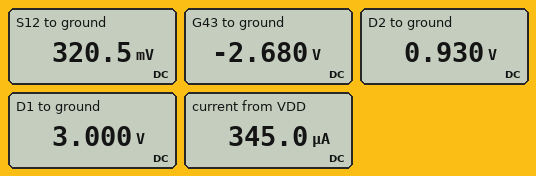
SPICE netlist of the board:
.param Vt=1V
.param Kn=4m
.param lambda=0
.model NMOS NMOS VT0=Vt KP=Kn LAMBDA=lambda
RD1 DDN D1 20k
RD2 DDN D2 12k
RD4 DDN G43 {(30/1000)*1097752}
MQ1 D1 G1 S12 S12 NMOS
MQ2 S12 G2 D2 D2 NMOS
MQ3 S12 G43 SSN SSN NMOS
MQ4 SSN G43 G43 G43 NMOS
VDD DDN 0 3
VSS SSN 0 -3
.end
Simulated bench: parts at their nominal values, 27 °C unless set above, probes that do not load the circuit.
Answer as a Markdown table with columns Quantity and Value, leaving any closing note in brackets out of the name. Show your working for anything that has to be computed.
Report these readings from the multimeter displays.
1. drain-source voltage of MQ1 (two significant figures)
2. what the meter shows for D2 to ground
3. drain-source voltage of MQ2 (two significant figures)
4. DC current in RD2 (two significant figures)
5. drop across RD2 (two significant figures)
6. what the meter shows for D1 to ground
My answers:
| Quantity | Value |
|---|---|
| drain-source voltage of MQ1 | 3 V - 320.5 mV = 2.7 V |
| what the meter shows for D2 to ground | 0.930 V |
| drain-source voltage of MQ2 | 320.5 mV - 930 mV = -610 mV |
| DC current in RD2 | (3 V - 930 mV) / 12 kΩ = 170 µA |
| drop across RD2 | 3 V - 930 mV = 2.1 V |
| what the meter shows for D1 to ground | 3.000 V |
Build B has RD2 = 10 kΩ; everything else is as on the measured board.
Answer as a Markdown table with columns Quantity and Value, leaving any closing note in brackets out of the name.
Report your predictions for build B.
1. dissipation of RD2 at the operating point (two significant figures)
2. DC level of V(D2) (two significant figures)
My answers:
| Quantity | Value |
|---|---|
| dissipation of RD2 at the operating point | 300 µW |
| DC level of V(D2) | 1.3 V |
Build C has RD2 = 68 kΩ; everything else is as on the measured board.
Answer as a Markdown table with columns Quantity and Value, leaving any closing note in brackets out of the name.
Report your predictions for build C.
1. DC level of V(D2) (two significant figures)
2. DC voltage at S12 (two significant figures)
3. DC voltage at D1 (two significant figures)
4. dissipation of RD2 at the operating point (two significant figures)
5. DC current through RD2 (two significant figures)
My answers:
| Quantity | Value |
|---|---|
| DC level of V(D2) | -220 mV |
| DC voltage at S12 | -280 mV |
| DC voltage at D1 | 500 mV |
| dissipation of RD2 at the operating point | 150 µW |
| DC current through RD2 | 47 µA |
